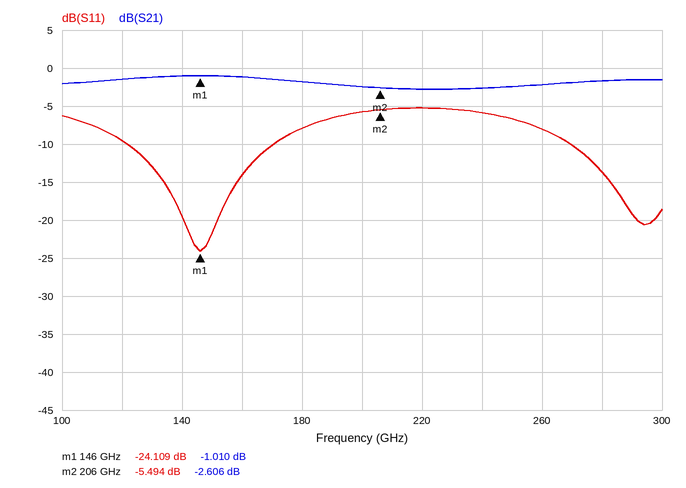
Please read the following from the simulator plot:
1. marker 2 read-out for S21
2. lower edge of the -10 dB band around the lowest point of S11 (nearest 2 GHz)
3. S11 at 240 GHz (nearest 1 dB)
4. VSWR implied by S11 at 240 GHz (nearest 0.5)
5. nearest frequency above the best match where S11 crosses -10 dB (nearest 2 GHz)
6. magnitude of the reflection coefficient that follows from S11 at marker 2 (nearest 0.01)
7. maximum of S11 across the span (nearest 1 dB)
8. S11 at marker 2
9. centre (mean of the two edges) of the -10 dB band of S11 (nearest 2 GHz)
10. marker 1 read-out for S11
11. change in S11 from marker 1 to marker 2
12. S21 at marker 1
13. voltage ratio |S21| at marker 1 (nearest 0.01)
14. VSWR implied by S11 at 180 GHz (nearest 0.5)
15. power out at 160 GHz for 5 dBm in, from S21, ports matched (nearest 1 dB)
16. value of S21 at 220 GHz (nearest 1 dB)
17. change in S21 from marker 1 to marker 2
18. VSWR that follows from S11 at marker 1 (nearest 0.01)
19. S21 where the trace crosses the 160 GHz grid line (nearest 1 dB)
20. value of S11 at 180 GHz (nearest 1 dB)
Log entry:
-2.606 dB
122 GHz
-6 dB
3.0
170 GHz
0.53
-5 dB
-5.494 dB
146 GHz
-24.109 dB
18.615 dB
-1.010 dB
0.89
2.5
4 dBm
-3 dB
-1.596 dB
1.13
-1 dB
-8 dB
